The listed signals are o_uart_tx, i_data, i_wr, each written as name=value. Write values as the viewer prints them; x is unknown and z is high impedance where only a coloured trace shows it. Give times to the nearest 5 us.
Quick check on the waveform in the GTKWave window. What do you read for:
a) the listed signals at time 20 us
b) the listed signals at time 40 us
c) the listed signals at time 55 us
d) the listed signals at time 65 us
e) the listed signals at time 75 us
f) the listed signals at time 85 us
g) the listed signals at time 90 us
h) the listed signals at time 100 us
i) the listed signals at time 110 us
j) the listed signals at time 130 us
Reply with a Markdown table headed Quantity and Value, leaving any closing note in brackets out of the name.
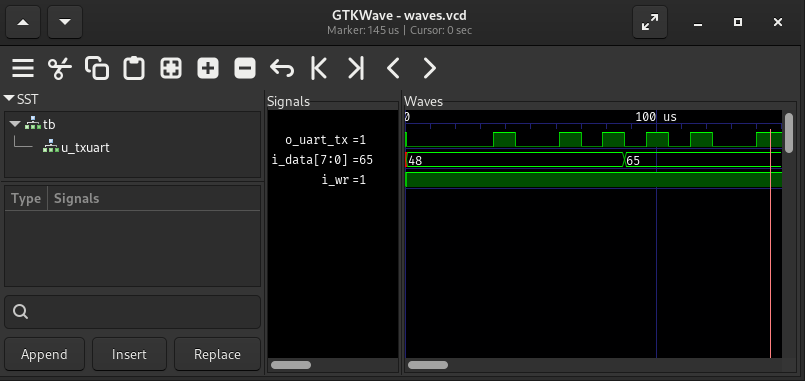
| Quantity | Value |
|---|---|
| the listed signals at time 20 us | o_uart_tx=0, i_data=48, i_wr=1 |
| the listed signals at time 40 us | o_uart_tx=1, i_data=48, i_wr=1 |
| the listed signals at time 55 us | o_uart_tx=0, i_data=48, i_wr=1 |
| the listed signals at time 65 us | o_uart_tx=1, i_data=48, i_wr=1 |
| the listed signals at time 75 us | o_uart_tx=0, i_data=48, i_wr=1 |
| the listed signals at time 85 us | o_uart_tx=1, i_data=48, i_wr=1 |
| the listed signals at time 90 us | o_uart_tx=0, i_data=65, i_wr=1 |
| the listed signals at time 100 us | o_uart_tx=1, i_data=65, i_wr=1 |
| the listed signals at time 110 us | o_uart_tx=0, i_data=65, i_wr=1 |
| the listed signals at time 130 us | o_uart_tx=0, i_data=65, i_wr=1 |
